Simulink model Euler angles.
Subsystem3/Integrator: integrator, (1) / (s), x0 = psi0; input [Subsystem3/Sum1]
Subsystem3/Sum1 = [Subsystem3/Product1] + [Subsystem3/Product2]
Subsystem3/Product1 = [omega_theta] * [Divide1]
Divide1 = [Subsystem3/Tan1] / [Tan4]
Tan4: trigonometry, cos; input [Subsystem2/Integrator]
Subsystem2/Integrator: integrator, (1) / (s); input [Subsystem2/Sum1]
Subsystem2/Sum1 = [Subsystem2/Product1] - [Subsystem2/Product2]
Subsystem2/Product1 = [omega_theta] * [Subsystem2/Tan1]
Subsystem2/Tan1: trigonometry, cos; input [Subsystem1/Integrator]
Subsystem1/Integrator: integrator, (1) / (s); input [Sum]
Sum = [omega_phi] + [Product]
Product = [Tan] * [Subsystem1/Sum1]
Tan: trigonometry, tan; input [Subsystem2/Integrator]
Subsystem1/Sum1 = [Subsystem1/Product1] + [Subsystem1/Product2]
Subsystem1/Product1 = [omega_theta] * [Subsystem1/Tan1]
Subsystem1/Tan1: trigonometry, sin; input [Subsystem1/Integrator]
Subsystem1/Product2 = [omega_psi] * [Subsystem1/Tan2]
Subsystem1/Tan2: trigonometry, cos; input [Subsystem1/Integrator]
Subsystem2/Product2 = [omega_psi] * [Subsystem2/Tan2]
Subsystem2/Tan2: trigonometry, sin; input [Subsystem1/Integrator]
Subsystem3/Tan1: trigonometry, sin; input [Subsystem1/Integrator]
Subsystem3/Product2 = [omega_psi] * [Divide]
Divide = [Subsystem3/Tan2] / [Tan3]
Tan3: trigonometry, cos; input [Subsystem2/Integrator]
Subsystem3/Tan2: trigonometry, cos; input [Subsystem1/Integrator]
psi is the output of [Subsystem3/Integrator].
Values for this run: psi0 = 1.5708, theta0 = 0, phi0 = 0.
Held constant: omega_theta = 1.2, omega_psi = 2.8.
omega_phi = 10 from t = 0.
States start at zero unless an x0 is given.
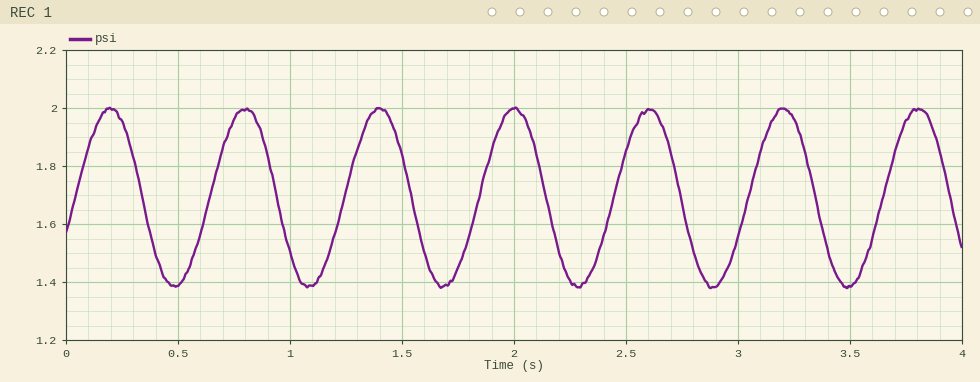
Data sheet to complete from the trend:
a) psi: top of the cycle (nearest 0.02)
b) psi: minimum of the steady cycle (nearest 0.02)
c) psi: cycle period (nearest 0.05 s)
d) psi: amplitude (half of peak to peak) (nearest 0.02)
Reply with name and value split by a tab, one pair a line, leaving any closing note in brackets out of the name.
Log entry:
psi: top of the cycle	2.00
psi: minimum of the steady cycle	1.38
psi: cycle period	0.60 s
psi: amplitude (half of peak to peak)	0.30
